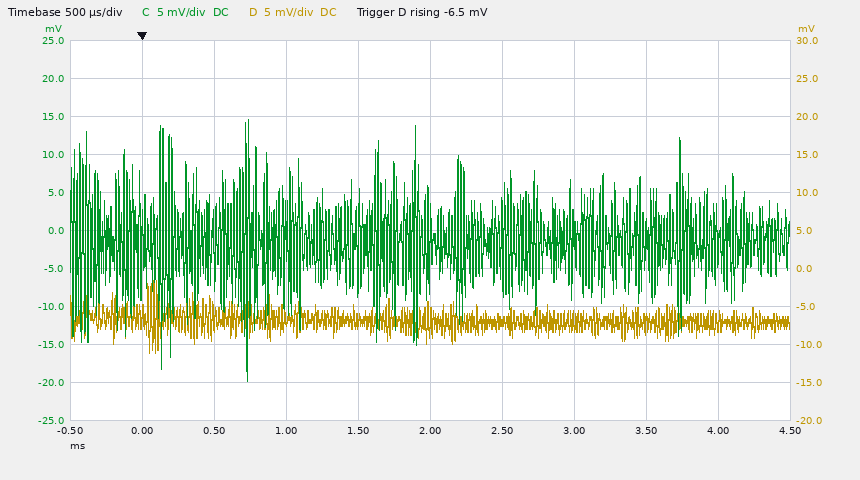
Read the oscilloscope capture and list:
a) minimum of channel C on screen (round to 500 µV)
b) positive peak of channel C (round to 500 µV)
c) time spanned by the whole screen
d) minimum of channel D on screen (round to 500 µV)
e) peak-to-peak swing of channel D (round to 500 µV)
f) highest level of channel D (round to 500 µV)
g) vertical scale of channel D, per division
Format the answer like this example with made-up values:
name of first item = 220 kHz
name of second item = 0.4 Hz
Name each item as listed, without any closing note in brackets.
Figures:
minimum of channel C on screen = -19.5 mV
positive peak of channel C = 14.5 mV
time spanned by the whole screen = 5 ms
minimum of channel D on screen = -11.0 mV
peak-to-peak swing of channel D = 9.5 mV
highest level of channel D = -1.5 mV
vertical scale of channel D, per division = 5 mV
